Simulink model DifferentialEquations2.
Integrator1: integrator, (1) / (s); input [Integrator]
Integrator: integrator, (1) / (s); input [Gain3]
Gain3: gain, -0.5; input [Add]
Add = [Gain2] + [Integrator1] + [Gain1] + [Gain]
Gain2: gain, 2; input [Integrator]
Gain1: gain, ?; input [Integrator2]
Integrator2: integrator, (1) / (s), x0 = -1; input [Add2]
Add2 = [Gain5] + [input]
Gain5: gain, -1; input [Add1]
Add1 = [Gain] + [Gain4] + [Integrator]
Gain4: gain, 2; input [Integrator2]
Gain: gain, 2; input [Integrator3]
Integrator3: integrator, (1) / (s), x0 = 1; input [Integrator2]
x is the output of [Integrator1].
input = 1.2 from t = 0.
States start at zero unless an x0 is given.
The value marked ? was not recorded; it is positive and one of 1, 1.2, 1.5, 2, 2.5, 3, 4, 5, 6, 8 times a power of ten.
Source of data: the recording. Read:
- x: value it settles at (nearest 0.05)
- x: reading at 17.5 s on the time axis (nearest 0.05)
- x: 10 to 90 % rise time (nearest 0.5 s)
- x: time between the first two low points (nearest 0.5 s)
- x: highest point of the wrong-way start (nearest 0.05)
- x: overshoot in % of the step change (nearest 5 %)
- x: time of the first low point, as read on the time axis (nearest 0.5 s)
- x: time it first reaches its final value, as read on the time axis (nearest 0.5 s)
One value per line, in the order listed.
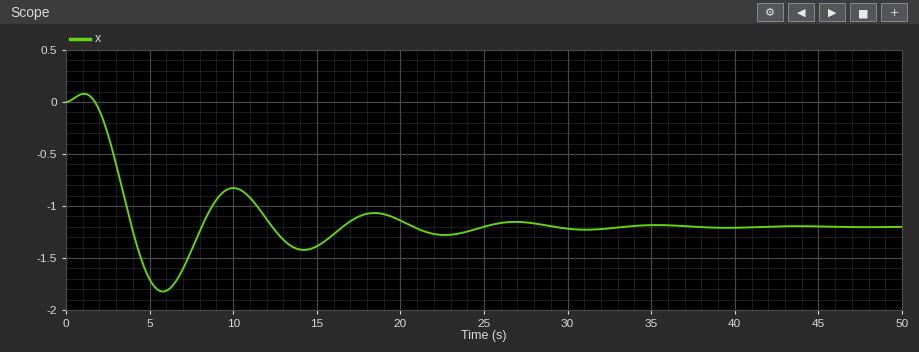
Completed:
-1.20
-1.10
1.5 s
8.5 s
0.10
50 %
6.0 s
4.0 s
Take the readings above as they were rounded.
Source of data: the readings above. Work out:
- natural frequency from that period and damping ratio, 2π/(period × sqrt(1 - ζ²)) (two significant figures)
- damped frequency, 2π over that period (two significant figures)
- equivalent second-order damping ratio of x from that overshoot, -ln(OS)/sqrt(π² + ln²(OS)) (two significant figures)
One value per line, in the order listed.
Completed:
0.76 rad/s
0.74 rad/s
0.22
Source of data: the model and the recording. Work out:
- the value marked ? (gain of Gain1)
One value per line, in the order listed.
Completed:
3
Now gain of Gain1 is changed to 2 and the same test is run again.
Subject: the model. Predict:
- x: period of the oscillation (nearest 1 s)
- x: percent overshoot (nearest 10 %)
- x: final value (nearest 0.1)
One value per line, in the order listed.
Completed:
9 s
40 %
-1.2
